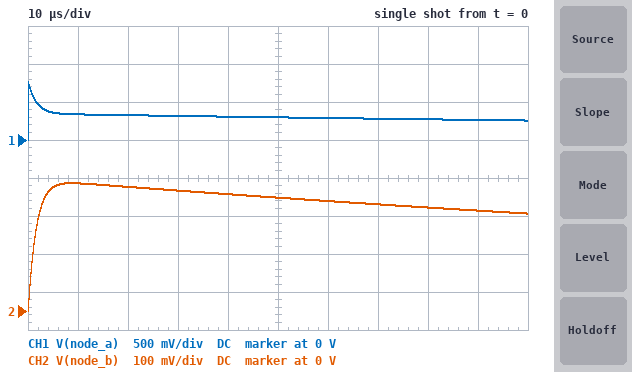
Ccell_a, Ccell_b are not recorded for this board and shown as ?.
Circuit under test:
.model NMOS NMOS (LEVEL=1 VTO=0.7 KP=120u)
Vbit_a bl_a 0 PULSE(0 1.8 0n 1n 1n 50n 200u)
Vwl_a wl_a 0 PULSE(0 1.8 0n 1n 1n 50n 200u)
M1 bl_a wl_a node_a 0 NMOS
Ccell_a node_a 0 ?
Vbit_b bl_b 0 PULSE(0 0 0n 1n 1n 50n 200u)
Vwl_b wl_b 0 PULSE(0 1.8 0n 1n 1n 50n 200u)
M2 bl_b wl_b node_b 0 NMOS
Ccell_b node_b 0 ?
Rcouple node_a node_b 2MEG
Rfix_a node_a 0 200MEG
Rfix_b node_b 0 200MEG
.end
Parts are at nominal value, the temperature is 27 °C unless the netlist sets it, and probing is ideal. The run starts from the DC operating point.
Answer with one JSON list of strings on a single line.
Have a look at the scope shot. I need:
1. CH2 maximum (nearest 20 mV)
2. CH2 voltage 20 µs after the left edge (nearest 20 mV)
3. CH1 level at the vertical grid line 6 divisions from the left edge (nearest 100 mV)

["340 mV", "320 mV", "300 mV"]
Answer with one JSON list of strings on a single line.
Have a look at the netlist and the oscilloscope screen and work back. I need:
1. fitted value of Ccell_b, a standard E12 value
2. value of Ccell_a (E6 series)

["1.8 pF", "1.5 pF"]
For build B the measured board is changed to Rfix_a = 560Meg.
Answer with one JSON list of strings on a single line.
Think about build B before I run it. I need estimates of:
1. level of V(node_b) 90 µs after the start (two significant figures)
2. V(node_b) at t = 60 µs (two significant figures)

["290 mV", "310 mV"]
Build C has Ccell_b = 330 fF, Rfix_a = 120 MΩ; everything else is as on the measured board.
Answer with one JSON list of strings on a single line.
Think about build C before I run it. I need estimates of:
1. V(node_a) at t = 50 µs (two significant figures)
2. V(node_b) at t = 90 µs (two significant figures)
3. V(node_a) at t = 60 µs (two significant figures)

["430 mV", "320 mV", "400 mV"]
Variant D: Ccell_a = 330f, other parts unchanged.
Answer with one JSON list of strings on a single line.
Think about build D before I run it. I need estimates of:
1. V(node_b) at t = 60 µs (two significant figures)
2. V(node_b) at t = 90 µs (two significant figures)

["120 mV", "100 mV"]
